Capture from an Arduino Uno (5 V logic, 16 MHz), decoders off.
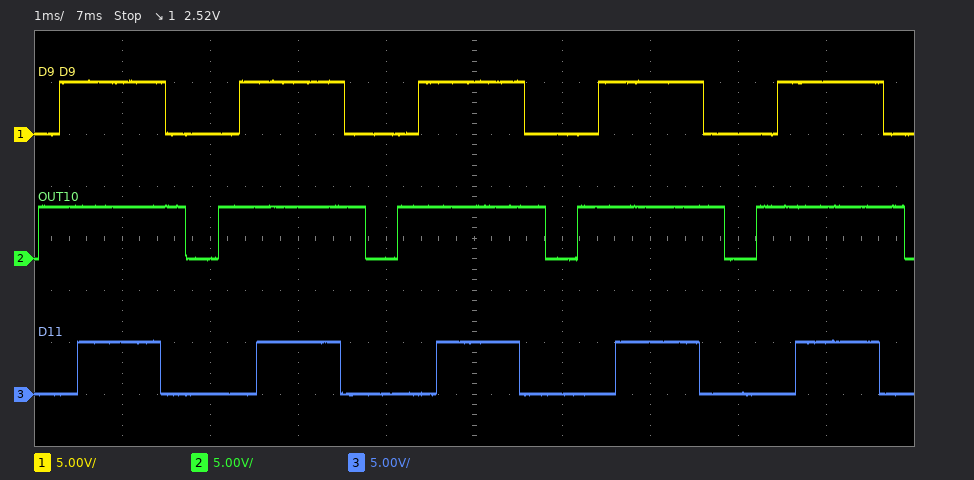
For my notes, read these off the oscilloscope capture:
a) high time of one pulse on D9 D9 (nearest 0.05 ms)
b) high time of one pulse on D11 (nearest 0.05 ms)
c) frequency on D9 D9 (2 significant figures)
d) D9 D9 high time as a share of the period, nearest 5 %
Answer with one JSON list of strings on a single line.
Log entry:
["1.20 ms", "0.95 ms", "490 Hz", "60 %"]
